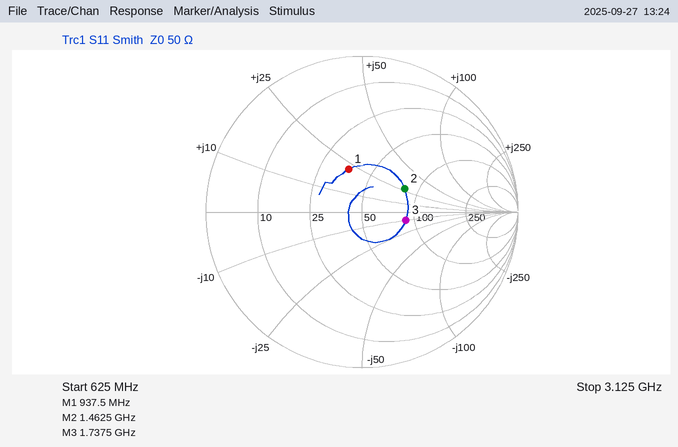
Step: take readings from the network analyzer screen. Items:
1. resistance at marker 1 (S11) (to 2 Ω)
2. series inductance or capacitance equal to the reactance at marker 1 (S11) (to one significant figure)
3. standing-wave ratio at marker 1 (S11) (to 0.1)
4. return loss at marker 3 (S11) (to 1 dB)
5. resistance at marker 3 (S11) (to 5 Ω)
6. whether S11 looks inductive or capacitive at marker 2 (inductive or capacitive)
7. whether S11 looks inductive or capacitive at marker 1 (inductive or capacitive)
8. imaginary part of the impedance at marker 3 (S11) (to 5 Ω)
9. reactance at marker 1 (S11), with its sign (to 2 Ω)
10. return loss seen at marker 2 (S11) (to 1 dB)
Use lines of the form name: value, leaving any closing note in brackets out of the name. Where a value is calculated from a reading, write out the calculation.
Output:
resistance at marker 1 (S11): 36 Ω
series inductance or capacitance equal to the reactance at marker 1 (S11): L = 22 Ω/(2π × 937.5 MHz) ≈ 4 nH
standing-wave ratio at marker 1 (S11): 1.8
return loss at marker 3 (S11): 11 dB
resistance at marker 3 (S11): 90 Ω
whether S11 looks inductive or capacitive at marker 2: inductive
whether S11 looks inductive or capacitive at marker 1: inductive
imaginary part of the impedance at marker 3 (S11): -10 Ω
reactance at marker 1 (S11), with its sign: +22 Ω
return loss seen at marker 2 (S11): 10 dB
